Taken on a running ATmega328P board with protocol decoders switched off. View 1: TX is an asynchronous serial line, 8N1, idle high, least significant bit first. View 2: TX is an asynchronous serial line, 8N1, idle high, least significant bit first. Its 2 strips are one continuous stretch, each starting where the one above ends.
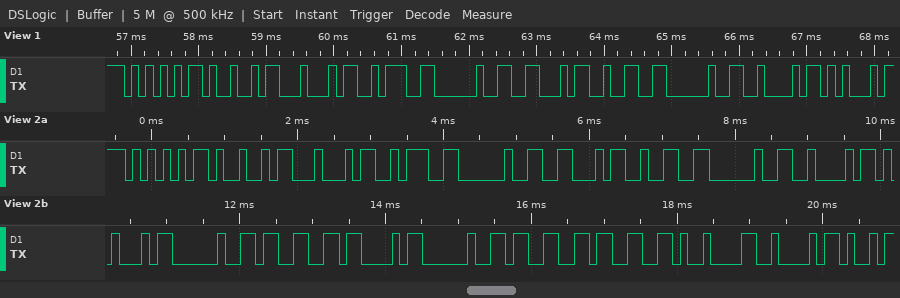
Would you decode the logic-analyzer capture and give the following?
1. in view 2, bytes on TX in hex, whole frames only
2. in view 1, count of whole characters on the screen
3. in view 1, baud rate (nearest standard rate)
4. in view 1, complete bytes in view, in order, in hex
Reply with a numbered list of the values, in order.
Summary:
1. 0x55 0x49 0x44 0x3A 0x20 0x46 0x32 0x20 0x42 0x45 0x20 0x33 0x43 0x20 0x33 0x33 0x09 0x42
2. 10
3. 9600 baud
4. 0x55 0x49 0x44 0x3A 0x20 0x46 0x32 0x20 0x42 0x45
